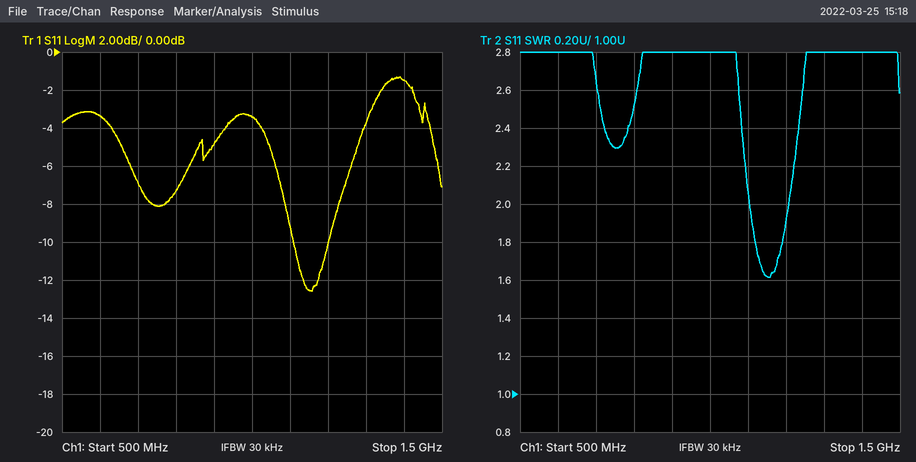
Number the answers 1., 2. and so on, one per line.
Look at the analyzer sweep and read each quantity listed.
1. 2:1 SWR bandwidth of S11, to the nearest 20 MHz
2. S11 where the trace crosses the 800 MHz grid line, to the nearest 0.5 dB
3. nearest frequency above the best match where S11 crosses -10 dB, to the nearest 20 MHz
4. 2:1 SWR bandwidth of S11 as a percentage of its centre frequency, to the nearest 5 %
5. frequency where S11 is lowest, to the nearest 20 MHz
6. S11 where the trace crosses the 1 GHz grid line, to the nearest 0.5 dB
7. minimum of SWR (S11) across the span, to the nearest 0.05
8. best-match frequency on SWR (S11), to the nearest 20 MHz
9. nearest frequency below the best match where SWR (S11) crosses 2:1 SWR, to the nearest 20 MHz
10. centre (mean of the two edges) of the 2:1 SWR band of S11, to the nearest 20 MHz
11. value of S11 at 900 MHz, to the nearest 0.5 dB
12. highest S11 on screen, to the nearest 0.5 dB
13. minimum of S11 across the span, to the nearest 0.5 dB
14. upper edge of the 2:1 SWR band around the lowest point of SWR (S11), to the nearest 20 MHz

1. 100 MHz
2. -7.5 dB
3. 1.20 GHz
4. 10 %
5. 1.16 GHz
6. -3.5 dB
7. 1.60
8. 1.16 GHz
9. 1.10 GHz
10. 1.16 GHz
11. -5.0 dB
12. -1.5 dB
13. -12.5 dB
14. 1.20 GHz
